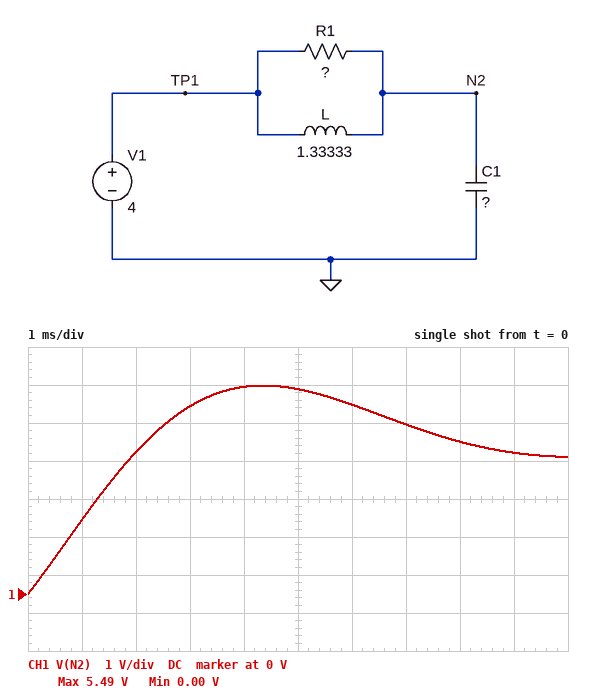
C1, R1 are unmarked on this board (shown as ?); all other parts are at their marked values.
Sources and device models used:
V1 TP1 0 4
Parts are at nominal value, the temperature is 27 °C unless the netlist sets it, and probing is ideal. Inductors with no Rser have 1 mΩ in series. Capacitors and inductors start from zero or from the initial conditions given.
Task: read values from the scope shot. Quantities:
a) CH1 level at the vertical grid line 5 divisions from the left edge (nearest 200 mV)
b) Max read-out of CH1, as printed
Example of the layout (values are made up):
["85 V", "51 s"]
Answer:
["5.4 V", "5.49 V"]
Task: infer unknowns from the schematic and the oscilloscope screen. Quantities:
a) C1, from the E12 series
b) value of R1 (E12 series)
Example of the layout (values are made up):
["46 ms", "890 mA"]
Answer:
["2.2 µF", "1 kΩ"]
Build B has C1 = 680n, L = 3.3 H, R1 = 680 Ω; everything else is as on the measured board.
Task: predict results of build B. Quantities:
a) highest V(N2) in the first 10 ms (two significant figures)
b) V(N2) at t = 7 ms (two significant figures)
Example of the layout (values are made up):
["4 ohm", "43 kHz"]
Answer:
["4.3 V", "4.1 V"]
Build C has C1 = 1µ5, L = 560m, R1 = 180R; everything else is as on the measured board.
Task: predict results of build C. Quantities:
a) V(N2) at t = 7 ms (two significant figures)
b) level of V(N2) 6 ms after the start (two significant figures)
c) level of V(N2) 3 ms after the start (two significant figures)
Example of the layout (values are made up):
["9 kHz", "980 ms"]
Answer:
["4.0 V", "4.1 V", "4.2 V"]
